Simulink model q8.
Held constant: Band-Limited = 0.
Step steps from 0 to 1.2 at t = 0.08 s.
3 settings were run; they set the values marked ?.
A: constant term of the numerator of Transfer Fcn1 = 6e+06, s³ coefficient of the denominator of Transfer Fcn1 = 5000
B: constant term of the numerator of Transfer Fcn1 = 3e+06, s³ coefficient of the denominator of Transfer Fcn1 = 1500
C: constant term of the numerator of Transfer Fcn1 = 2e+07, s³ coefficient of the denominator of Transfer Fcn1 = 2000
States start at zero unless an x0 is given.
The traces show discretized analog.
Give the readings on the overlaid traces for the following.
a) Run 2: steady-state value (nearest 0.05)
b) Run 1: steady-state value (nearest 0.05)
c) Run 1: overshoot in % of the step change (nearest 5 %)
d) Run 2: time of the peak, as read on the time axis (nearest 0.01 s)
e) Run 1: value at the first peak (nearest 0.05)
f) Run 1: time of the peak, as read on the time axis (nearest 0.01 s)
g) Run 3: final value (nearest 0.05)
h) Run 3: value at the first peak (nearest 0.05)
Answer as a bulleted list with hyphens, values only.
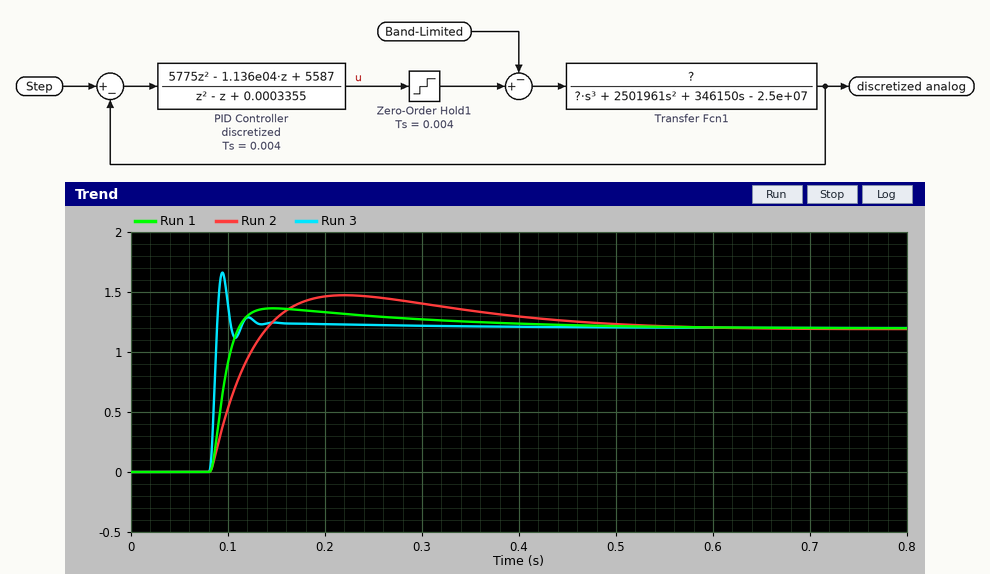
- 1.20
- 1.20
- 15 %
- 0.22 s
- 1.35
- 0.15 s
- 1.20
- 1.65
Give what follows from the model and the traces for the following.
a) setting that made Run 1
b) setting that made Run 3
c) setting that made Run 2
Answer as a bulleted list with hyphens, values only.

- A
- C
- B
